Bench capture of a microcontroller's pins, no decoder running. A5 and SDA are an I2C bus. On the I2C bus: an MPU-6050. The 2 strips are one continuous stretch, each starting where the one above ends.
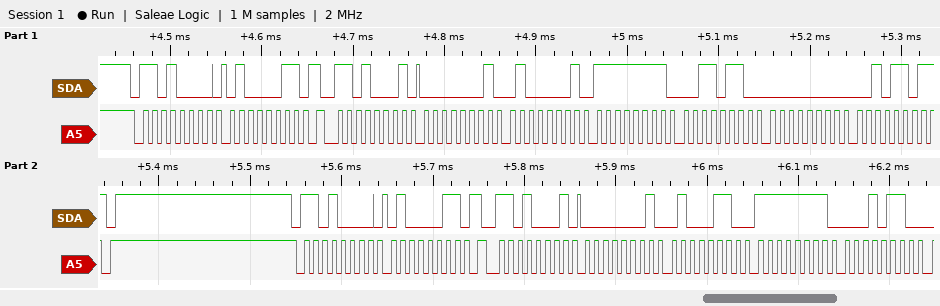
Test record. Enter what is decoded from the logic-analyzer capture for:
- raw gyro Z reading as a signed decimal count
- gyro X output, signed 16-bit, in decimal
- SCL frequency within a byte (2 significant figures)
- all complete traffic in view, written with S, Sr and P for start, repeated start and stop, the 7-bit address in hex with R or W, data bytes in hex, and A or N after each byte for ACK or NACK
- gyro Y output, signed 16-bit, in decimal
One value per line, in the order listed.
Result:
45
321
100 kHz
S 68W A 43 A Sr 68R A 01 A 41 A FF A 36 A 00 A 2D N P S 68W A 43 A Sr 68R A 01 A 46 A FF A 16 A
-202
